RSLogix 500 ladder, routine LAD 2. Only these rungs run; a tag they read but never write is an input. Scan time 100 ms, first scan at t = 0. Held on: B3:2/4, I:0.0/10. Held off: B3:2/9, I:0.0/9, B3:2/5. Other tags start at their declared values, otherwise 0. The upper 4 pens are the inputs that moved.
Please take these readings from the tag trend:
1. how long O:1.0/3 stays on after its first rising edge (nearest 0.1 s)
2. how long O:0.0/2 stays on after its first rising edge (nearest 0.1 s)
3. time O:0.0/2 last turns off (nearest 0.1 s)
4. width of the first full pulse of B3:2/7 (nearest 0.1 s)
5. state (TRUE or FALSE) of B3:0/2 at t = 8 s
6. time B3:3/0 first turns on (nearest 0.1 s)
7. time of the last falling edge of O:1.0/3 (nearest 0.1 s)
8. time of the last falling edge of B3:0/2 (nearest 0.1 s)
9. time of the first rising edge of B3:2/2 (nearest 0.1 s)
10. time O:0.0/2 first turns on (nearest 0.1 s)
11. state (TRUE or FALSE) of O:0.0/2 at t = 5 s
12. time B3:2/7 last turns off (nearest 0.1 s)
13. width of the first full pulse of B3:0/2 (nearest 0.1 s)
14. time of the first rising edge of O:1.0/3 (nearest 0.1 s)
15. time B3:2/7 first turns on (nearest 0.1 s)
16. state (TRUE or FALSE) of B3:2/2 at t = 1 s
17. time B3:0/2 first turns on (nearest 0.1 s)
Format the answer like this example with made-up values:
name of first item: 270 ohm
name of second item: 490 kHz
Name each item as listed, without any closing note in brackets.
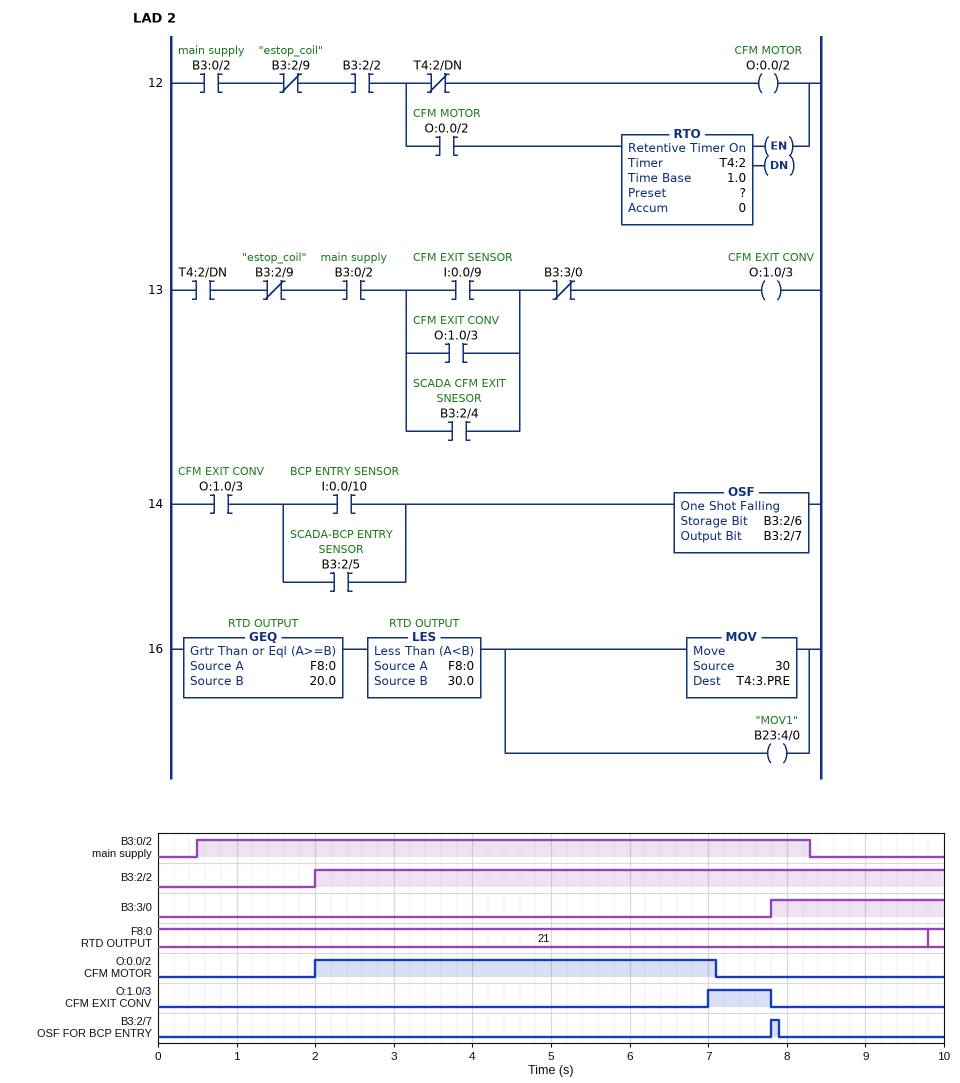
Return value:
how long O:1.0/3 stays on after its first rising edge: 0.8 s
how long O:0.0/2 stays on after its first rising edge: 5.1 s
time O:0.0/2 last turns off: 7.1 s
width of the first full pulse of B3:2/7: 0.1 s
state (TRUE or FALSE) of B3:0/2 at t = 8 s: TRUE
time B3:3/0 first turns on: 7.8 s
time of the last falling edge of O:1.0/3: 7.8 s
time of the last falling edge of B3:0/2: 8.3 s
time of the first rising edge of B3:2/2: 2.0 s
time O:0.0/2 first turns on: 2.0 s
state (TRUE or FALSE) of O:0.0/2 at t = 5 s: TRUE
time B3:2/7 last turns off: 7.9 s
width of the first full pulse of B3:0/2: 7.8 s
time of the first rising edge of O:1.0/3: 7.0 s
time B3:2/7 first turns on: 7.8 s
state (TRUE or FALSE) of B3:2/2 at t = 1 s: FALSE
time B3:0/2 first turns on: 0.5 s
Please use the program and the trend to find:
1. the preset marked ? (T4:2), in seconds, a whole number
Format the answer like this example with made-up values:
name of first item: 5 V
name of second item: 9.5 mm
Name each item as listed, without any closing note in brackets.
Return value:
the preset marked ? (T4:2), in seconds, a whole number: 5 s
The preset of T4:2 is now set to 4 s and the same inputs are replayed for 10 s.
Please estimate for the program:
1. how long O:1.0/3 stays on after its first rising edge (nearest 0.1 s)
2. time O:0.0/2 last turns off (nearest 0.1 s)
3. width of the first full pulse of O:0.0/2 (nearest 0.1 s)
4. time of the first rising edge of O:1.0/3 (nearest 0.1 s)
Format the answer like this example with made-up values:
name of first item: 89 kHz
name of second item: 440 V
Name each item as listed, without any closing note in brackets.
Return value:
how long O:1.0/3 stays on after its first rising edge: 1.8 s
time O:0.0/2 last turns off: 6.1 s
width of the first full pulse of O:0.0/2: 4.1 s
time of the first rising edge of O:1.0/3: 6.0 s
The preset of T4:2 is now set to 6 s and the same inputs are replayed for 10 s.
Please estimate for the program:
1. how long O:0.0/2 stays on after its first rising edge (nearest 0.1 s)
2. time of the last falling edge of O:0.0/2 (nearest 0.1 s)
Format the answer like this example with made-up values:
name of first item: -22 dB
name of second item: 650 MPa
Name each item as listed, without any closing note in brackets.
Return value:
how long O:0.0/2 stays on after its first rising edge: 6.1 s
time of the last falling edge of O:0.0/2: 8.1 s
